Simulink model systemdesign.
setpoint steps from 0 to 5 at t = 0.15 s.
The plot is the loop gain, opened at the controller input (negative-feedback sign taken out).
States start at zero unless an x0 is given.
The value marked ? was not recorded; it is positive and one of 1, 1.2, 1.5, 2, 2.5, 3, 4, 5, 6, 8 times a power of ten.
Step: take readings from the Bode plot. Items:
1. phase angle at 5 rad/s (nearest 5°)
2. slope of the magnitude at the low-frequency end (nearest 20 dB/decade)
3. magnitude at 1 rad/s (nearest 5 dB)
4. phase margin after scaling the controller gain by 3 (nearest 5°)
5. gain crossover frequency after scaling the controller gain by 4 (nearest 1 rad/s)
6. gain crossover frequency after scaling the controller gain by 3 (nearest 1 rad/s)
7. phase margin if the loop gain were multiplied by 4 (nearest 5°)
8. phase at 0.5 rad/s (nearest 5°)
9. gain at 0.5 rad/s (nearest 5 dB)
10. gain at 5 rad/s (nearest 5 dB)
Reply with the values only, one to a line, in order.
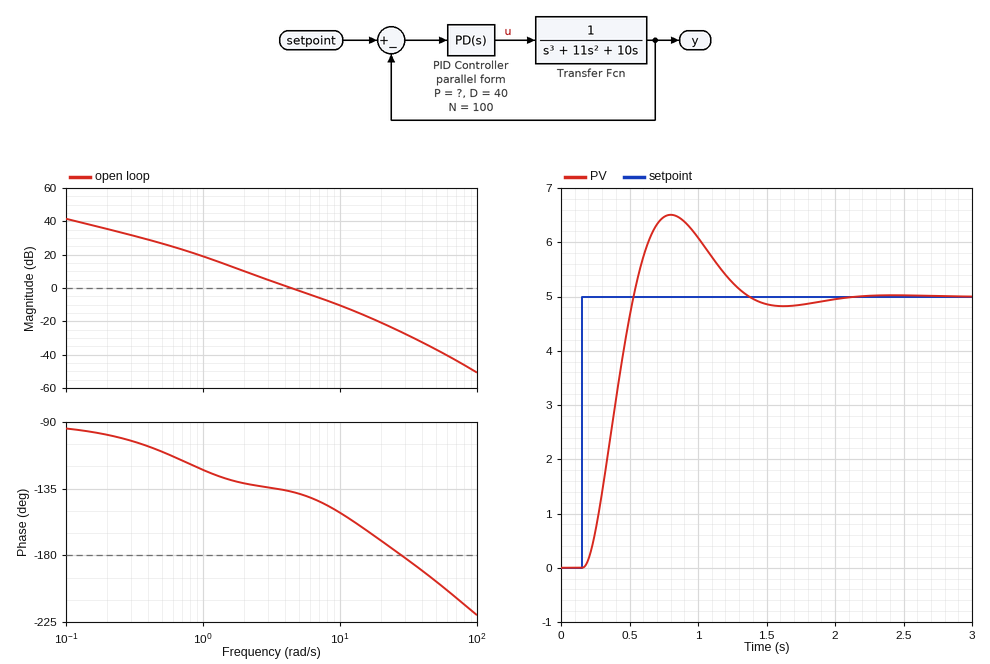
-140°
-20 dB/decade
20 dB
30°
11 rad/s
9 rad/s
25°
-110°
25 dB
0 dB
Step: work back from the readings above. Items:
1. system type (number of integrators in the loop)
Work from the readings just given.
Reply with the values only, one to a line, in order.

1
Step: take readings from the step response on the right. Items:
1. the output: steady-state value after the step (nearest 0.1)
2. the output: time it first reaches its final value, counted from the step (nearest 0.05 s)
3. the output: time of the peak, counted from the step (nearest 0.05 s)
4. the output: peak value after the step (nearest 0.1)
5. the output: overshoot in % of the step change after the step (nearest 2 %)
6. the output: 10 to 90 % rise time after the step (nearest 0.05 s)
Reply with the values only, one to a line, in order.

5.0
0.40 s
0.65 s
6.5
30 %
0.25 s
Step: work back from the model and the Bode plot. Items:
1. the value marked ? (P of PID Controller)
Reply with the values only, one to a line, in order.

120
